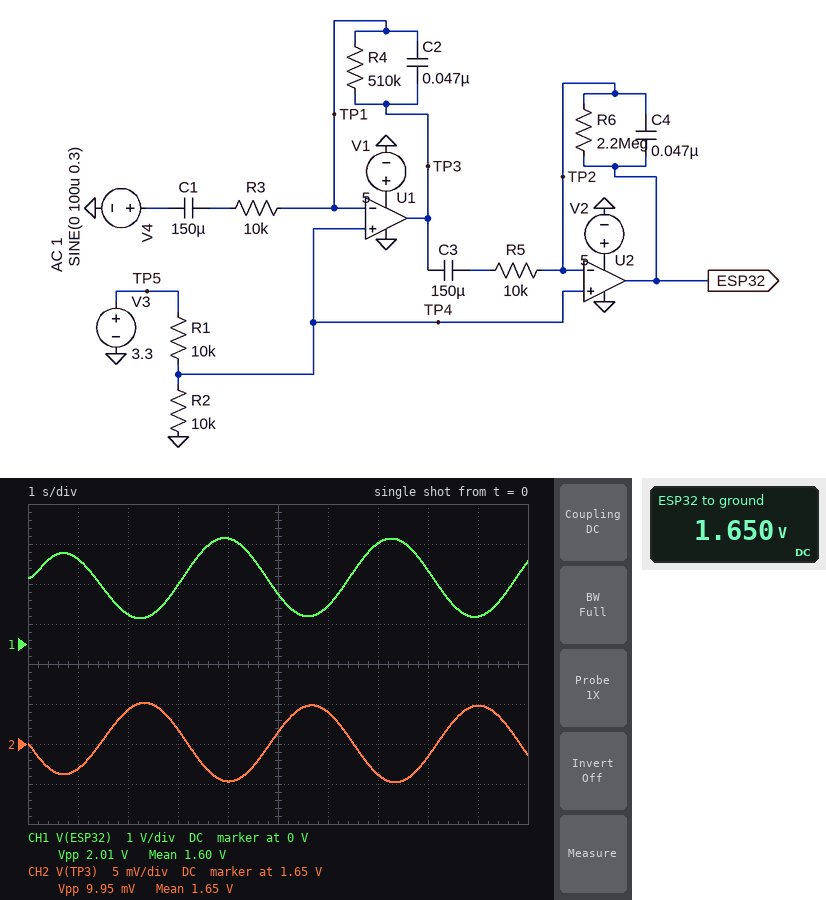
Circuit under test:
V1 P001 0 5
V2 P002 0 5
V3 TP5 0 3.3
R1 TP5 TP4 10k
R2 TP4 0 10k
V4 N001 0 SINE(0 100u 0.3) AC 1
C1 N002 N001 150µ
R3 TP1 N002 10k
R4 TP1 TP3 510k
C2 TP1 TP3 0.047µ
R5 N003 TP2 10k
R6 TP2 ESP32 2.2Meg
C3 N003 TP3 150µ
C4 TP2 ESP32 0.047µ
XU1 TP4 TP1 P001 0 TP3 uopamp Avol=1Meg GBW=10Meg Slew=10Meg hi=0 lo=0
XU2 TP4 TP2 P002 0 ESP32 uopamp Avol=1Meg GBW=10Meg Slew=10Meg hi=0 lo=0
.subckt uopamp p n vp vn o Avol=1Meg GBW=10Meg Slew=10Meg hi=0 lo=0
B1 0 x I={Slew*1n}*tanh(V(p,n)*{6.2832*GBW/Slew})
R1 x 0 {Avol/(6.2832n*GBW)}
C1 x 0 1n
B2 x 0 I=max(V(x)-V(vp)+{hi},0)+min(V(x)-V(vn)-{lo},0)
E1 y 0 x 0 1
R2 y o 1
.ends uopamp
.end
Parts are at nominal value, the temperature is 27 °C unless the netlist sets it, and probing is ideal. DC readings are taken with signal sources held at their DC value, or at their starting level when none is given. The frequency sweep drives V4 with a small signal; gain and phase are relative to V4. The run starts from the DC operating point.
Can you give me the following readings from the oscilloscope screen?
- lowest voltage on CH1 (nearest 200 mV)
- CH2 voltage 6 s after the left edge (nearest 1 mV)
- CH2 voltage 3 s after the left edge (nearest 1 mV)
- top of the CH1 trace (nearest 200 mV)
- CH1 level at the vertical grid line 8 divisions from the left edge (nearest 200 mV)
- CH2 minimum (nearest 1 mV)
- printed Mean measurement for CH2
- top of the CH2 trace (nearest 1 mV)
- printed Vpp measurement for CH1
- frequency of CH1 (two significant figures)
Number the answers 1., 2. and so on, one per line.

1. 600 mV
2. 1.654 V
3. 1.652 V
4. 2.6 V
5. 1.8 V
6. 1.645 V
7. 1.65 V
8. 1.655 V
9. 2.01 V
10. 300 mHz
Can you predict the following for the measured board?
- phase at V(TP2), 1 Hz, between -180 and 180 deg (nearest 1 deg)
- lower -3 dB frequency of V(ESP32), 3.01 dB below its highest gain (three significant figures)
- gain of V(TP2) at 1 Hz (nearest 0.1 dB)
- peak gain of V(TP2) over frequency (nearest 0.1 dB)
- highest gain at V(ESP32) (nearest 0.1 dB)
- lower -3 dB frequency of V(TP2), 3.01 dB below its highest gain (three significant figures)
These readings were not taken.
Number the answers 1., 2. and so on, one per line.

1. 156 deg
2. 143 mHz
3. -40.7 dB
4. -39.8 dB
5. 80.2 dB
6. 143 mHz
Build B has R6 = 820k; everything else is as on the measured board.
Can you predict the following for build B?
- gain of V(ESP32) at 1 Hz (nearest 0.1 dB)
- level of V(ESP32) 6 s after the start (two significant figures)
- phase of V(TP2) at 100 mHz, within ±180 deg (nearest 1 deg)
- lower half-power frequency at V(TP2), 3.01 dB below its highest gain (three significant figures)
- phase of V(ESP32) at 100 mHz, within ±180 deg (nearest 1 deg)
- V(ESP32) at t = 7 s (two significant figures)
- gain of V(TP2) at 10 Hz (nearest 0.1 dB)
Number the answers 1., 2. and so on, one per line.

1. 72.0 dB
2. 1.4 V
3. -88 deg
4. 155 mHz
5. 91 deg
6. 2.0 V
7. -58.1 dB
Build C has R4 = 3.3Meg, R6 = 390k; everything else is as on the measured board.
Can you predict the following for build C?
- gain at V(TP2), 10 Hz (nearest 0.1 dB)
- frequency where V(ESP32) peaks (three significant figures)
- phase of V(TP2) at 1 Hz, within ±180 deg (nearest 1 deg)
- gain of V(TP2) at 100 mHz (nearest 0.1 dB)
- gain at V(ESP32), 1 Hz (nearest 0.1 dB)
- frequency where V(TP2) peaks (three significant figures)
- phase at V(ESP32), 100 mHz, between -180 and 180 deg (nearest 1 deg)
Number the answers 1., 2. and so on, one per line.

1. -58.3 dB
2. 398 mHz
3. 147 deg
4. -44.4 dB
5. 79.1 dB
6. 399 mHz
7. 87 deg
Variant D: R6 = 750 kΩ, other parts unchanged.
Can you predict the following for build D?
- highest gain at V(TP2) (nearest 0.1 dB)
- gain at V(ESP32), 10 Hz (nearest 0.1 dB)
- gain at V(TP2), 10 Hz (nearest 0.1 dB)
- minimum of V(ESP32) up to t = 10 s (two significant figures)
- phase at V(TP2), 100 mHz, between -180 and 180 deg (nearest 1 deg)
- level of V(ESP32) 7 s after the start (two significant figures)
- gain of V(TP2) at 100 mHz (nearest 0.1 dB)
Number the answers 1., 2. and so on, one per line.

1. -48.7 dB
2. 58.8 dB
3. -58.2 dB
4. 1.3 V
5. -88 deg
6. 2.0 V
7. -54.9 dB
